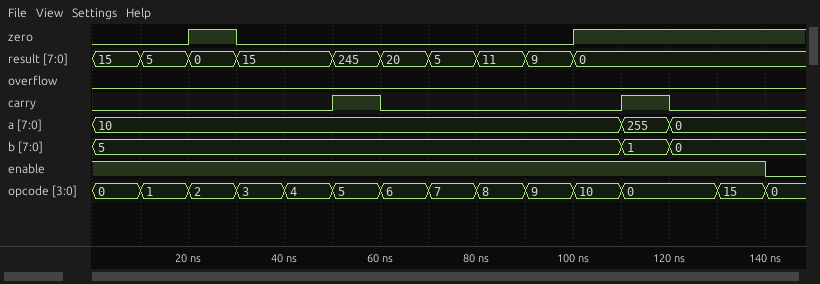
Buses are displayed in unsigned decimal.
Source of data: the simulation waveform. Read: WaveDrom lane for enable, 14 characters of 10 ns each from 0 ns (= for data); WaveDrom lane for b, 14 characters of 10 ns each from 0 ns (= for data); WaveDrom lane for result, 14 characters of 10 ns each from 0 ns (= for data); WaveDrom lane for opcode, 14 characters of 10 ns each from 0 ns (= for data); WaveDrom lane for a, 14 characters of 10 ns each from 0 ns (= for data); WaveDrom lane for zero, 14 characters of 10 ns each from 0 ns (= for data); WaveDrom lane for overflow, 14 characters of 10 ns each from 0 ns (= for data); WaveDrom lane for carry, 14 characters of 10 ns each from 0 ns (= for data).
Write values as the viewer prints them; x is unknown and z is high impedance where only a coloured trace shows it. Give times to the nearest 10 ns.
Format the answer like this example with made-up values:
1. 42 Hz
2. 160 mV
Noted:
1. {name: 'enable', wave: '1.............'}
2. {name: 'b', wave: '=..........==.', data: '5 1 0'}
3. {name: 'result', wave: '====.======...', data: '15 5 0 15 245 20 5 11 9 0'}
4. {name: 'opcode', wave: '============.=', data: '0 1 2 3 4 5 6 7 8 9 10 0 15'}
5. {name: 'a', wave: '=..........==.', data: '10 255 0'}
6. {name: 'zero', wave: '0.10......1...'}
7. {name: 'overflow', wave: '0.............'}
8. {name: 'carry', wave: '0....10....10.'}
